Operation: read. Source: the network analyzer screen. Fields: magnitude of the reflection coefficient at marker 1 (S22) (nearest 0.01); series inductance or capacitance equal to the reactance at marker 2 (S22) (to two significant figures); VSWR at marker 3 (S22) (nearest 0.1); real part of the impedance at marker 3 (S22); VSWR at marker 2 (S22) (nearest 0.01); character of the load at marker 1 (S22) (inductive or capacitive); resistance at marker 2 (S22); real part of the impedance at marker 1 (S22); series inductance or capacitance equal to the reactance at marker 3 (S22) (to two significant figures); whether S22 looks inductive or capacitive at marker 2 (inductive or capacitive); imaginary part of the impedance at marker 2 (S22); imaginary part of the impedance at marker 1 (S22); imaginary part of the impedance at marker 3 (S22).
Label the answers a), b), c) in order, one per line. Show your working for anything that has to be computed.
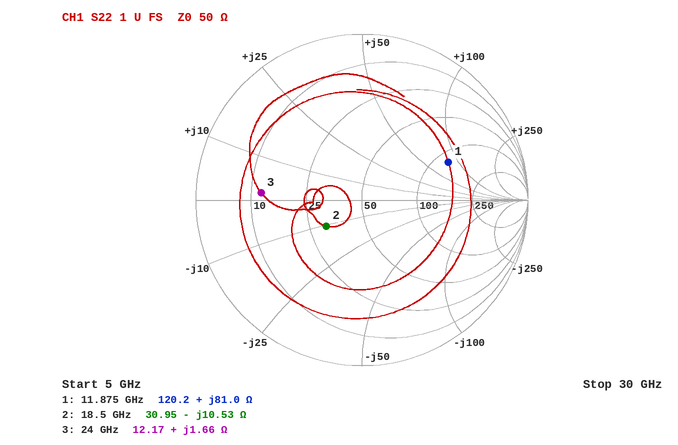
a) 0.57
b) C = 1/(2π × 18.5 GHz × 10.53 Ω) ≈ 817 fF, so 820 fF to two significant figures
c) 4.1
d) 12.17 Ω
e) 1.73
f) inductive
g) 30.95 Ω
h) 120.2 Ω
i) L = 1.66 Ω/(2π × 24 GHz) ≈ 11 pH
j) capacitive
k) -10.53 Ω
l) +81.0 Ω
m) +1.66 Ω
